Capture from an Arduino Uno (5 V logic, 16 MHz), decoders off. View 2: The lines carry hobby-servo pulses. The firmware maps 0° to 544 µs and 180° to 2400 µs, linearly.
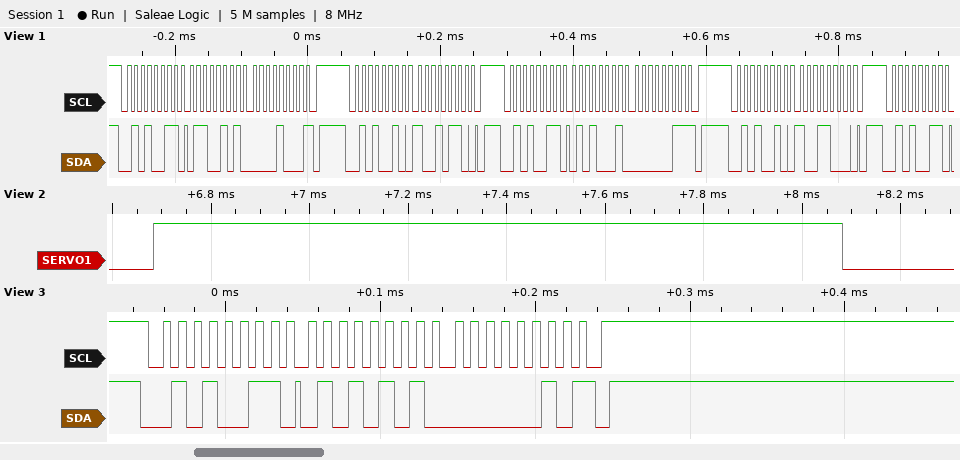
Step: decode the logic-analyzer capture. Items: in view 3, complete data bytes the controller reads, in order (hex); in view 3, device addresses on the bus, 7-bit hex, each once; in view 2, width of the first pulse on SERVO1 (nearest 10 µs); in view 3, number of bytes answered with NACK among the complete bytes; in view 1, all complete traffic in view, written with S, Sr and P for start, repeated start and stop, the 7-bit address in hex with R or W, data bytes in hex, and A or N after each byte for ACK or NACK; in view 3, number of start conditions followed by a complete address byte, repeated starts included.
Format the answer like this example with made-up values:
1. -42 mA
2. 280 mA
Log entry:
1. 55 02
2. 0x29
3. 1400 µs
4. 1
5. S 29R A 65 A 08 N P S 29W A 96 A P S 29R A 51 A 03 N P S 29W A 98 A P S 29R A
6. 1
